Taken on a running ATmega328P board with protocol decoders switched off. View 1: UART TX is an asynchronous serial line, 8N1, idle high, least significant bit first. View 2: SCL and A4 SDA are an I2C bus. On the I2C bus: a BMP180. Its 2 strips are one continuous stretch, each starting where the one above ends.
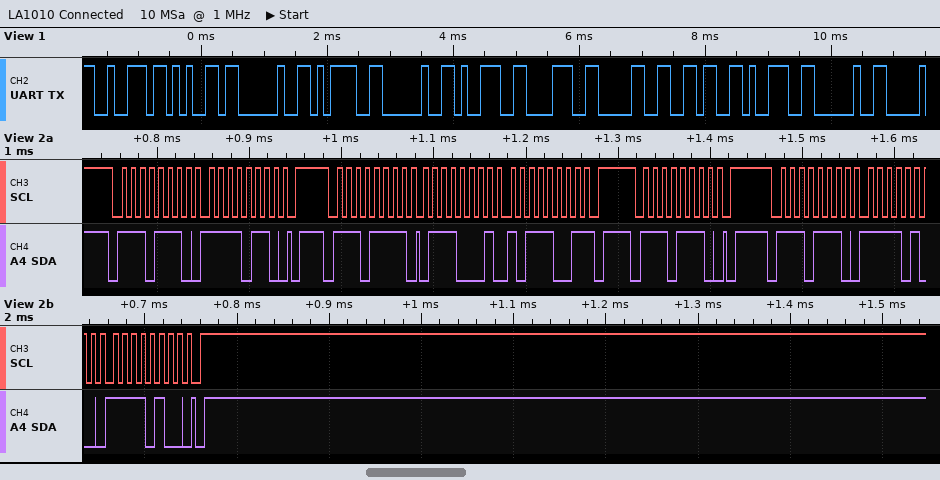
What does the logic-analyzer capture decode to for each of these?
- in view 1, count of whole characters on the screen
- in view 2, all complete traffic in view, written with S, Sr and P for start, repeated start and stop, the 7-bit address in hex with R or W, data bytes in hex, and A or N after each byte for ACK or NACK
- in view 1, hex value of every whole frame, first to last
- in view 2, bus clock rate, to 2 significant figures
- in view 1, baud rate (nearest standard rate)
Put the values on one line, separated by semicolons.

11; S 77W A F6 A P S 77R A 71 A B9 N P S 77W A P S 77W A F4 A F4 A P; 72 65 20 3D 20 39 38 30 36 39 20; 100 kHz; 9600 baud
